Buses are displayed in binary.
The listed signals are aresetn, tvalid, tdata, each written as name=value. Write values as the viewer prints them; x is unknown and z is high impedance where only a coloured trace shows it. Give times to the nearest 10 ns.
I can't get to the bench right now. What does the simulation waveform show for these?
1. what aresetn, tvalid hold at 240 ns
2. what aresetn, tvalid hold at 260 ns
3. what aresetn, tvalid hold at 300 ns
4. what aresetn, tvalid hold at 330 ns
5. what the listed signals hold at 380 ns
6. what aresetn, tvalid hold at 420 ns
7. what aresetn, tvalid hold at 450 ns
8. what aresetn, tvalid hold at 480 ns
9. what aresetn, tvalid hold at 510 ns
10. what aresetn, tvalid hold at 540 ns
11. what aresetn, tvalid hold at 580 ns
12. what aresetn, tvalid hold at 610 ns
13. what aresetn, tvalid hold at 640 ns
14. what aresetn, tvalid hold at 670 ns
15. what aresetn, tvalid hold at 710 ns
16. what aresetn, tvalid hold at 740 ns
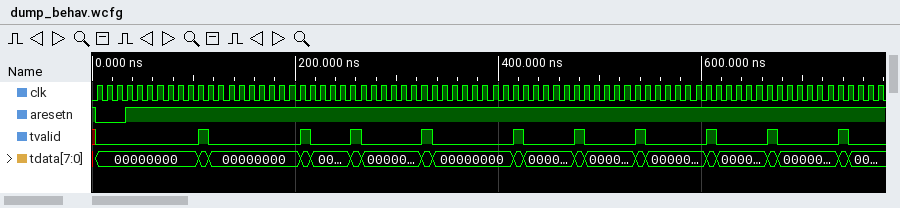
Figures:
aresetn=1, tvalid=0
aresetn=1, tvalid=1
aresetn=1, tvalid=0
aresetn=1, tvalid=1
aresetn=1, tvalid=0, tdata=00000000
aresetn=1, tvalid=1
aresetn=1, tvalid=0
aresetn=1, tvalid=1
aresetn=1, tvalid=0
aresetn=1, tvalid=1
aresetn=1, tvalid=0
aresetn=1, tvalid=1
aresetn=1, tvalid=0
aresetn=1, tvalid=1
aresetn=1, tvalid=0
aresetn=1, tvalid=1
